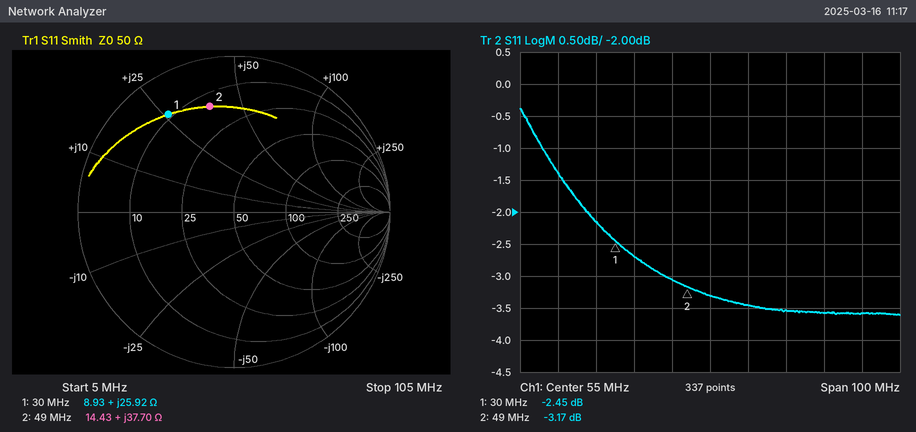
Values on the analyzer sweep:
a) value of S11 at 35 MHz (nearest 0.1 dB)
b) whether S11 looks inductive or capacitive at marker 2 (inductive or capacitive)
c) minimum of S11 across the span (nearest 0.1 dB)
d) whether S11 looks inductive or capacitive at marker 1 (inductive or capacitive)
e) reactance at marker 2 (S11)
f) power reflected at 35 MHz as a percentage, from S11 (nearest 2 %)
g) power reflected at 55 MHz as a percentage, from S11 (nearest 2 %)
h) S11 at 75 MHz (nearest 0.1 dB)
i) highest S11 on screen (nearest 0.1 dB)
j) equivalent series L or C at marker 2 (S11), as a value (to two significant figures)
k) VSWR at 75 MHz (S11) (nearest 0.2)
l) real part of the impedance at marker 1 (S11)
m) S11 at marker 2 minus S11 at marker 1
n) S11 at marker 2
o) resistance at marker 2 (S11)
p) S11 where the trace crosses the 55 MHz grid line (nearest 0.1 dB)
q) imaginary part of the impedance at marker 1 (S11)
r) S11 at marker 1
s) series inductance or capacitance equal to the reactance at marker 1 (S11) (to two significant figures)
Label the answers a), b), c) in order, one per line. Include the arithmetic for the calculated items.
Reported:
a) -2.7 dB
b) inductive
c) -3.6 dB
d) inductive
e) +37.70 Ω
f) 10^(-2.7/10) ≈ 54 %
g) 10^(-3.3/10) ≈ 46.8 %, so 46 % to the nearest 2 %
h) -3.5 dB
i) -0.4 dB
j) L = 37.7 Ω/(2π × 49 MHz) ≈ 122 nH, so 120 nH to two significant figures
k) |Γ| = 10^(-3.5/20) = 0.6683; VSWR = (1 + 0.6683)/(1 − 0.6683) ≈ 5.0
l) 8.93 Ω
m) -3.17 − (-2.45) = -0.72 dB
n) -3.17 dB
o) 14.43 Ω
p) -3.3 dB
q) +25.92 Ω
r) -2.45 dB
s) L = 25.92 Ω/(2π × 30 MHz) ≈ 138 nH, so 140 nH to two significant figures
